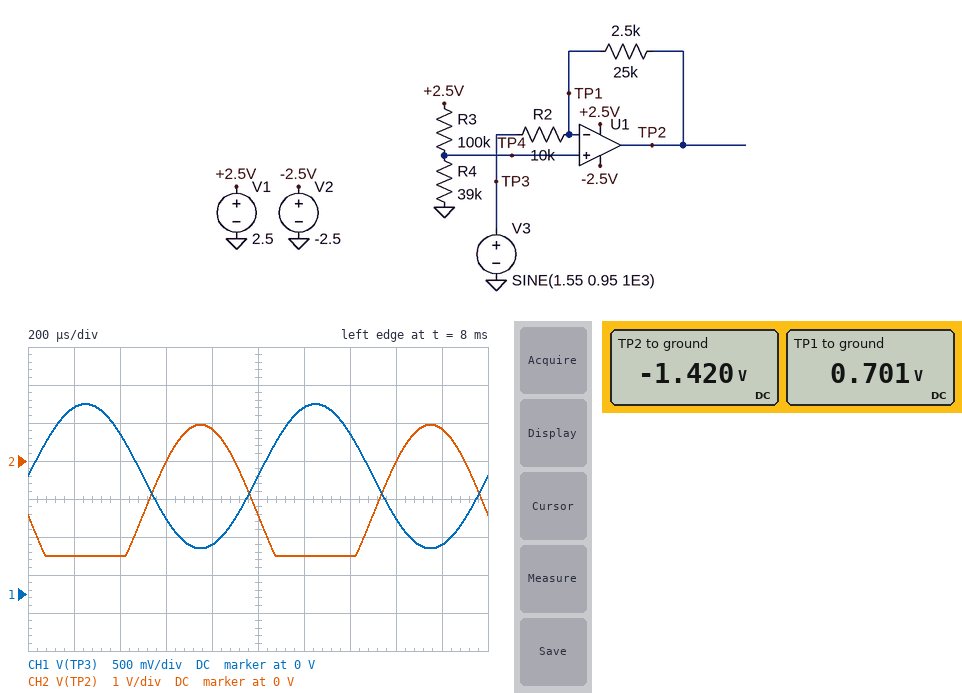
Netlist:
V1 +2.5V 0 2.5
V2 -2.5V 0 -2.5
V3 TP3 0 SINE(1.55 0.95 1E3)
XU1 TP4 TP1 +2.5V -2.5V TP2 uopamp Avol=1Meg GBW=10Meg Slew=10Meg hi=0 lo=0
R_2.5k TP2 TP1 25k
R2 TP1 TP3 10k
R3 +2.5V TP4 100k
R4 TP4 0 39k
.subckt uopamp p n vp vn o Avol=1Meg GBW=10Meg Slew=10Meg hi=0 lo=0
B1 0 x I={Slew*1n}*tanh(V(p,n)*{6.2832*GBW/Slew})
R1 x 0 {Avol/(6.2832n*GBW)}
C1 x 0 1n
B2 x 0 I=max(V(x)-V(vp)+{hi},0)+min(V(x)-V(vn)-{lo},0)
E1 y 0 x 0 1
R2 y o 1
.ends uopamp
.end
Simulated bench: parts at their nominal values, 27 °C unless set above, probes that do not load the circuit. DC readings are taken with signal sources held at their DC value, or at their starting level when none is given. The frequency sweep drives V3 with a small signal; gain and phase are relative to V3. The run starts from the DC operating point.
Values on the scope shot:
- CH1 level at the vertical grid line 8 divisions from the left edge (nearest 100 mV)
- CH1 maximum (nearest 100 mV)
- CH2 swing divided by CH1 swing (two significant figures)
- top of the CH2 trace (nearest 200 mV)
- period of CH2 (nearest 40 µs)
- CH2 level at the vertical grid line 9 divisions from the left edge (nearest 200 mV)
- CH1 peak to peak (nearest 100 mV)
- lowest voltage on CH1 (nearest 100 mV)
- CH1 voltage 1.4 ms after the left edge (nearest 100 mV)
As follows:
1.0 V
2.5 V
1.8
1.0 V
1.00 ms
800 mV
1.9 V
600 mV
2.1 V
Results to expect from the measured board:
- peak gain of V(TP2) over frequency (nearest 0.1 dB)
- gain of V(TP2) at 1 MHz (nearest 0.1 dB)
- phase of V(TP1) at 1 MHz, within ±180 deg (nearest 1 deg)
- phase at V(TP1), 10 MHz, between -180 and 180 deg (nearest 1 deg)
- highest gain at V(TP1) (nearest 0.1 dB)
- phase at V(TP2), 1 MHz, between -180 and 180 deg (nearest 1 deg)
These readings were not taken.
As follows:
8.0 dB
7.5 dB
71 deg
16 deg
-2.9 dB
161 deg
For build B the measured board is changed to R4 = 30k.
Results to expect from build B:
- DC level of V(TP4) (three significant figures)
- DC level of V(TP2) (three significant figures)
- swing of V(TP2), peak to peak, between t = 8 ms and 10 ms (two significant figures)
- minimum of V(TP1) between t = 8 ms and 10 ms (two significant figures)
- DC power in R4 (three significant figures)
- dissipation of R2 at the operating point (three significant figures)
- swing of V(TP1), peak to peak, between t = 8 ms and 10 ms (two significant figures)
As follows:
577 mV
-1.86 V
3.0 V
580 mV
11.1 µW
94.7 µW
490 mV
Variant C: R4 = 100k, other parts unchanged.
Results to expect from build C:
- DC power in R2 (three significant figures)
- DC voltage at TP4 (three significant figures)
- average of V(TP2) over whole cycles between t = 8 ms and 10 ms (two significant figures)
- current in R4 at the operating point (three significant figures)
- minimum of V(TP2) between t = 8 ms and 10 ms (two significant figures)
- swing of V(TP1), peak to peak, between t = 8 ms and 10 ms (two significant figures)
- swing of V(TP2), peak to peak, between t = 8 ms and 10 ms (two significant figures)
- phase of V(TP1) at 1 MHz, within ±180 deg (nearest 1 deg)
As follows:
9.00 µW
1.25 V
460 mV
12.5 µA
-1.9 V
110 mV
4.4 V
71 deg
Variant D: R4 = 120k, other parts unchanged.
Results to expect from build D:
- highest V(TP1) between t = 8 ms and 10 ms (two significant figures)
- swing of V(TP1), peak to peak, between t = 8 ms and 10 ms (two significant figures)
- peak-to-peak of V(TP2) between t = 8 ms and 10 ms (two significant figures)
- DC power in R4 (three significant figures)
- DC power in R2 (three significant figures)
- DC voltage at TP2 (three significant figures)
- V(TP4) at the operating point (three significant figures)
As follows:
1.4 V
220 mV
4.0 V
15.5 µW
3.47 µW
898 mV
1.36 V
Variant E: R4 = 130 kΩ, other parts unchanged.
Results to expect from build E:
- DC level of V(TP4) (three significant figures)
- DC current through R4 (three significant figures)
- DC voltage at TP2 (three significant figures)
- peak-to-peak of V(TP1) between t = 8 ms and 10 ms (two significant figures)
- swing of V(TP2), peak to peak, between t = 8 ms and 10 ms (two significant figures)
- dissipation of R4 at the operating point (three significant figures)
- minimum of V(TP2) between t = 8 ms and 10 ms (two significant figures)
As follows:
1.41 V
10.9 µA
1.07 V
270 mV
3.8 V
15.4 µW
-1.3 V
